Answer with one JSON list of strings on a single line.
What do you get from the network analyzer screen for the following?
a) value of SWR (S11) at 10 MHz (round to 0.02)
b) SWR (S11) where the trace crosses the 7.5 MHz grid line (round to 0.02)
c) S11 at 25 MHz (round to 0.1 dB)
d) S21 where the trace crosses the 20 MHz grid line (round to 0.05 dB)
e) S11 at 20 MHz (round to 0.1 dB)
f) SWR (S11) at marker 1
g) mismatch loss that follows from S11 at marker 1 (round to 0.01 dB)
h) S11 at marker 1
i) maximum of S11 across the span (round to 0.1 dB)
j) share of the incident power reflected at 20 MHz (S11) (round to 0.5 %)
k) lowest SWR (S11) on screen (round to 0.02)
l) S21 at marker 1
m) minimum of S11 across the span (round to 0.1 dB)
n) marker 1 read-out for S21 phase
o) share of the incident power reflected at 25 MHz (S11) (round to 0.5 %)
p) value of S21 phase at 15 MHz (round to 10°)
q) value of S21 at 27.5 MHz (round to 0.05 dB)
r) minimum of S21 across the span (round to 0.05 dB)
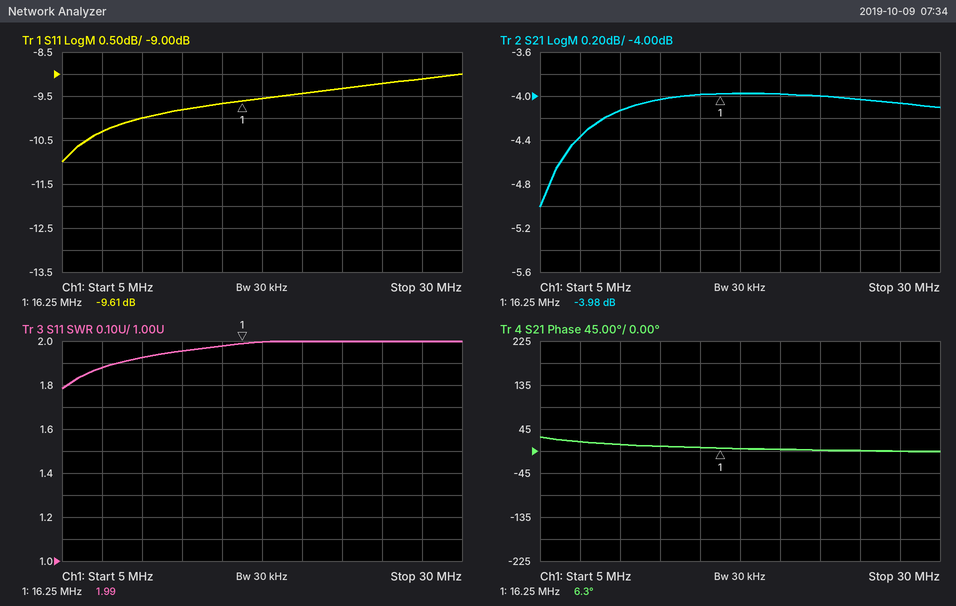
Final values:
["1.92", "1.88", "-9.2 dB", "-4.00 dB", "-9.4 dB", "1.99", "0.50 dB", "-9.61 dB", "-9.0 dB", "11.5 %", "1.78", "-3.98 dB", "-11.0 dB", "6.3°", "12.0 %", "10°", "-4.05 dB", "-5.00 dB"]
